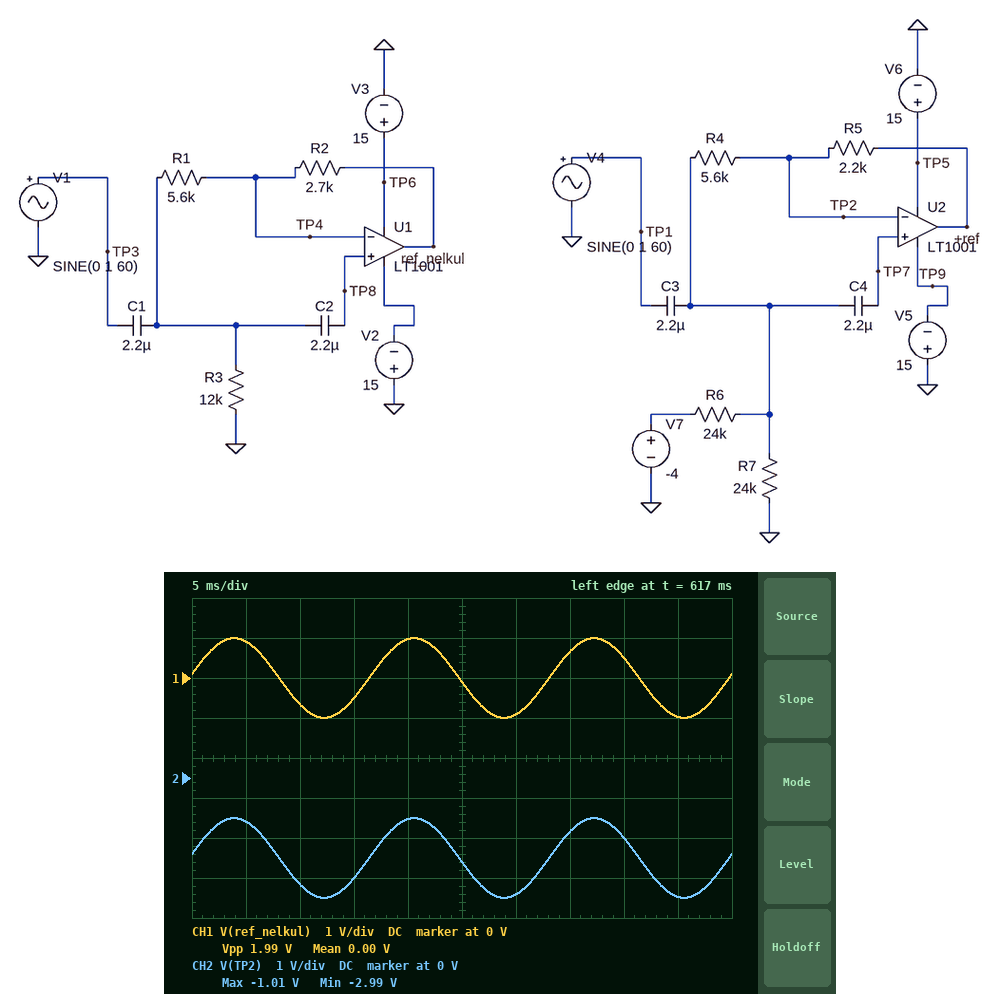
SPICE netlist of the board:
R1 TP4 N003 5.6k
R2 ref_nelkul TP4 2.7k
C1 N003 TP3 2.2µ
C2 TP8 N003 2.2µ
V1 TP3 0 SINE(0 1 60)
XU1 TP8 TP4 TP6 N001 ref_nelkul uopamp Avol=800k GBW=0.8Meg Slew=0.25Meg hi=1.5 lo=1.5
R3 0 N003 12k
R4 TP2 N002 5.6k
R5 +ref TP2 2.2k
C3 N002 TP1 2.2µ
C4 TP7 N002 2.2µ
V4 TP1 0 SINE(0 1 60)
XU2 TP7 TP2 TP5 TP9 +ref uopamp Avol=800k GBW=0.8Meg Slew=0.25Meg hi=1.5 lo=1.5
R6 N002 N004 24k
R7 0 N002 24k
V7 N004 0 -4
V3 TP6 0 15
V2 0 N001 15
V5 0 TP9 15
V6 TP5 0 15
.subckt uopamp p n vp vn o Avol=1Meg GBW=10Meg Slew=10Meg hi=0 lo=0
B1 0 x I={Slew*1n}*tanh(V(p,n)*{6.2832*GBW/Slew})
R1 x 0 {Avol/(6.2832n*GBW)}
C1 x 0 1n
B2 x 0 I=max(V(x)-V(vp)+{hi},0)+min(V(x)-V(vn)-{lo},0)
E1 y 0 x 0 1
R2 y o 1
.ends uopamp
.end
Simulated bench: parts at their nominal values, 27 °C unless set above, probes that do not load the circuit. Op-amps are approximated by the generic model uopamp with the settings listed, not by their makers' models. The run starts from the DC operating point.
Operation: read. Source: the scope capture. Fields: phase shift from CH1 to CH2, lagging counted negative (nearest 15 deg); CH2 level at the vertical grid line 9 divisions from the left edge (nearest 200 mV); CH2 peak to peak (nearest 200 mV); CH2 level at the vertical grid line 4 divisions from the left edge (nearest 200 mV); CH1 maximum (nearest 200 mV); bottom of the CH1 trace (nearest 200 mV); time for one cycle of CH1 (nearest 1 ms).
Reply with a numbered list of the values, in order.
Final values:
1. 0 deg
2. -3.0 V
3. 2.0 V
4. -1.0 V
5. 1.0 V
6. -1.0 V
7. 17 ms
